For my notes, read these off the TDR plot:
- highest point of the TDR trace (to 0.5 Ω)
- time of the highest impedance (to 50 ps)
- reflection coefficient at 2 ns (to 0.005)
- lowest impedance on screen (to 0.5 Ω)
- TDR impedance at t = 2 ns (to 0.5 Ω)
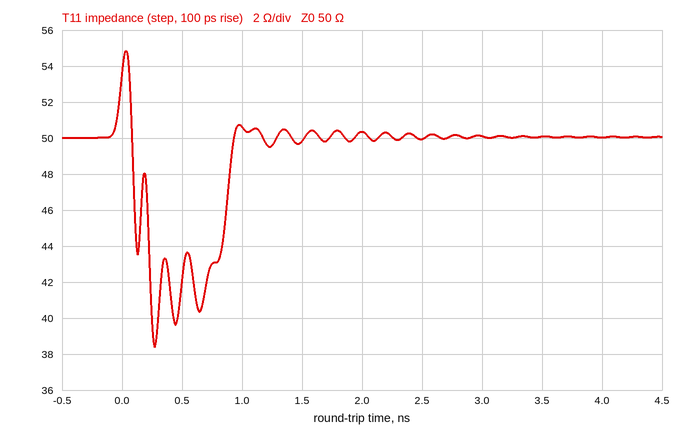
55.0 Ω
50 ps
+0.005
38.5 Ω
50.5 Ω
